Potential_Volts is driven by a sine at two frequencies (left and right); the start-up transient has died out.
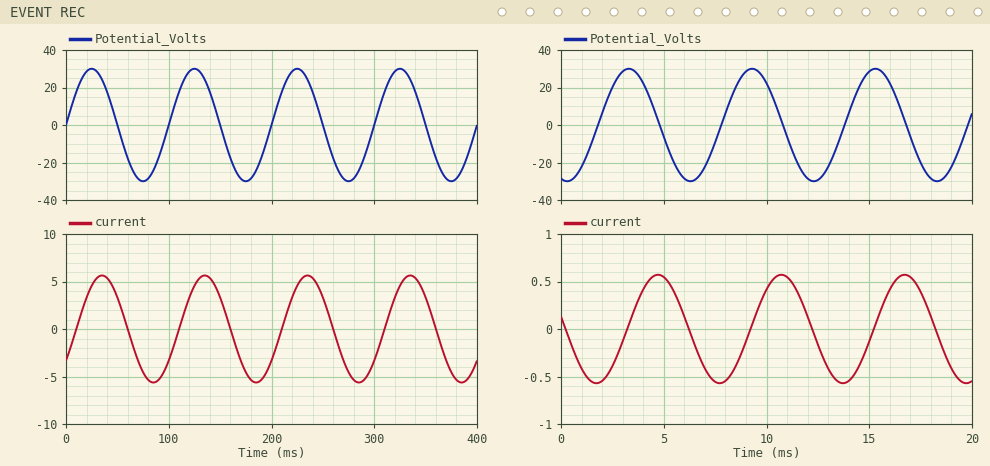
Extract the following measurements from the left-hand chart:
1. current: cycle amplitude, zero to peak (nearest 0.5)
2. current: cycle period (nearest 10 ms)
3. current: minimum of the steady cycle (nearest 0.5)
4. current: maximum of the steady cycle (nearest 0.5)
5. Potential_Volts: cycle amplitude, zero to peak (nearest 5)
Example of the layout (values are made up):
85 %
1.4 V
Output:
5.5
100 ms
-5.5
5.5
30
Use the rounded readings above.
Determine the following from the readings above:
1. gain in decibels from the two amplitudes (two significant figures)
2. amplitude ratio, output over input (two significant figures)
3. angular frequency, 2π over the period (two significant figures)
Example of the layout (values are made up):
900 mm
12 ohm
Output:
-15 dB
0.18
0.063 rad/ms
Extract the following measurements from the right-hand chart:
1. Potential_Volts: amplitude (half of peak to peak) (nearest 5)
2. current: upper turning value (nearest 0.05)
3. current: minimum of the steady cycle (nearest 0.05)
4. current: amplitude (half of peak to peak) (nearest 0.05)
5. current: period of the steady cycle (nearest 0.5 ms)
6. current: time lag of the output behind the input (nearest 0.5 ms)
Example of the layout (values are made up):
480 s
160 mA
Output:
30
0.55
-0.55
0.55
6.0 ms
1.5 ms
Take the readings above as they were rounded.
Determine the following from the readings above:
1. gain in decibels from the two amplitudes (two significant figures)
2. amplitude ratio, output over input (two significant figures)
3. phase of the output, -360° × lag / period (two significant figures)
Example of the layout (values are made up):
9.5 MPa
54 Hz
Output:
-35 dB
0.018
-90°
